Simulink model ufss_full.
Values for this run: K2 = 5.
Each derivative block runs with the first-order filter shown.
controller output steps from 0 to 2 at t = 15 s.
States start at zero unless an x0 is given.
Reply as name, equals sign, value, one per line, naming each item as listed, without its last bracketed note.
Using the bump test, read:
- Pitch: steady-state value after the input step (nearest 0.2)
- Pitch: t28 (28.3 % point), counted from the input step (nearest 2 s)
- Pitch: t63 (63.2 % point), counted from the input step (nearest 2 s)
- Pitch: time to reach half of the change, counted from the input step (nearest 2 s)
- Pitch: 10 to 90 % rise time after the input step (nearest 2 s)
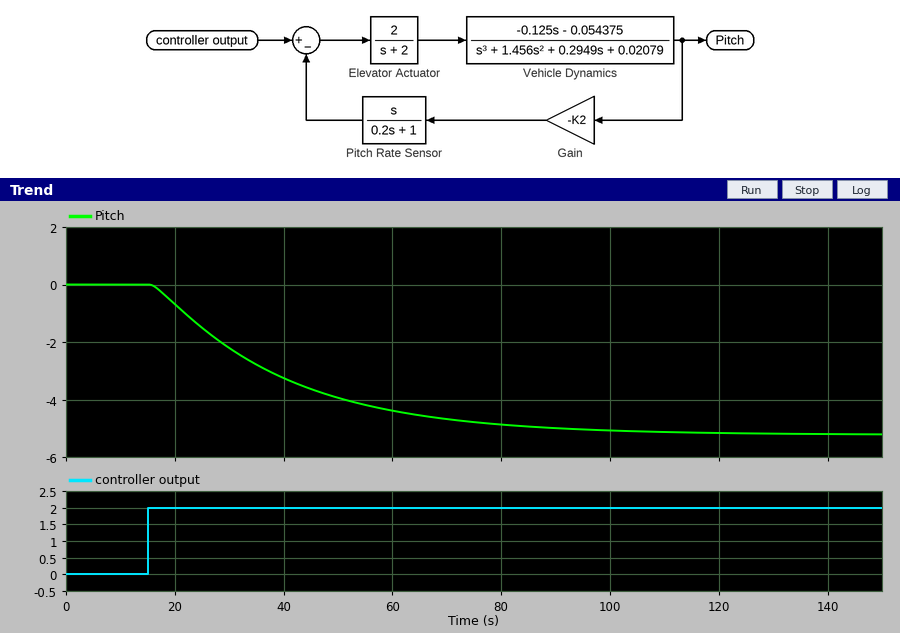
Pitch: steady-state value after the input step = -5.2
Pitch: t28 (28.3 % point), counted from the input step = 10 s
Pitch: t63 (63.2 % point), counted from the input step = 26 s
Pitch: time to reach half of the change, counted from the input step = 18 s
Pitch: 10 to 90 % rise time after the input step = 52 s
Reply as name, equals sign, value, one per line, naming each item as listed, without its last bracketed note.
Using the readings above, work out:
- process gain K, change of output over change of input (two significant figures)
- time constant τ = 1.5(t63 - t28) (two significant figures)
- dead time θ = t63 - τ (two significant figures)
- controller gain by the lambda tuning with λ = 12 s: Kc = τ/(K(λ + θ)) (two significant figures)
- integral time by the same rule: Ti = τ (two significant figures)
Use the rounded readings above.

process gain K, change of output over change of input = -2.6
time constant τ = 1.5(t63 - t28) = 24 s
dead time θ = t63 - τ = 2.0 s
controller gain by the lambda tuning with λ = 12 s: Kc = τ/(K(λ + θ)) = -0.66
integral time by the same rule: Ti = τ = 24 s
